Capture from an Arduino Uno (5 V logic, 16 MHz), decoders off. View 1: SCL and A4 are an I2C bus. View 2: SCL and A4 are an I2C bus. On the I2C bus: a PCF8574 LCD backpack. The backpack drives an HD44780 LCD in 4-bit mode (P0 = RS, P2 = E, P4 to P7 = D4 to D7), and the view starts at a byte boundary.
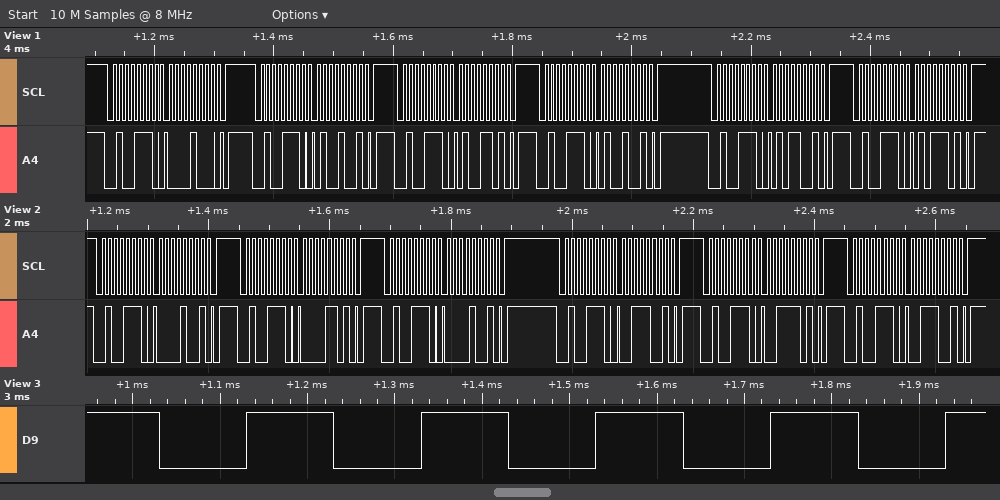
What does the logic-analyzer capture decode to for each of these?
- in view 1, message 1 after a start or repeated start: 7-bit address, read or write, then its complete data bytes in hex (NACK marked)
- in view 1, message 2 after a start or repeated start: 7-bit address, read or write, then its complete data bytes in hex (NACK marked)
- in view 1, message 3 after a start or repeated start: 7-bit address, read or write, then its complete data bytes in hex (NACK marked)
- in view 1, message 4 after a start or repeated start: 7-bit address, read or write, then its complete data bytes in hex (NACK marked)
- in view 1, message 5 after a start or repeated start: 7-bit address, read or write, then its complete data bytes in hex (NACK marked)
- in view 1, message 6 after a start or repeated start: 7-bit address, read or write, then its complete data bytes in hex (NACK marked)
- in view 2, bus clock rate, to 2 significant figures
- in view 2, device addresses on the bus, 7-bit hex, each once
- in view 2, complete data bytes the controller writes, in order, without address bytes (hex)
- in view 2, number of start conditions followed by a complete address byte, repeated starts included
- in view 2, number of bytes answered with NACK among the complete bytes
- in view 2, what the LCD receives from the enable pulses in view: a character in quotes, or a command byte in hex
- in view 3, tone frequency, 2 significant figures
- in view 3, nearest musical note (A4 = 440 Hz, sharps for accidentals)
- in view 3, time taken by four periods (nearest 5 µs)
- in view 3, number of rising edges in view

0x27 write: 08
0x27 write: 49
0x27 write: 4D
0x27 write: 49
0x27 write: 59
0x27 write: 5D
100 kHz
0x27
09 0D 09 39 3D 39
6
0
data 0x03
5.0 kHz
D#8
800 µs
5
